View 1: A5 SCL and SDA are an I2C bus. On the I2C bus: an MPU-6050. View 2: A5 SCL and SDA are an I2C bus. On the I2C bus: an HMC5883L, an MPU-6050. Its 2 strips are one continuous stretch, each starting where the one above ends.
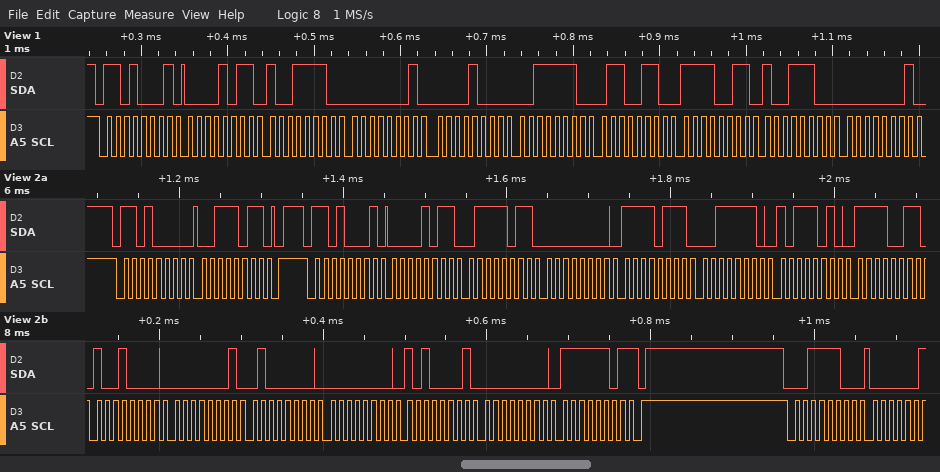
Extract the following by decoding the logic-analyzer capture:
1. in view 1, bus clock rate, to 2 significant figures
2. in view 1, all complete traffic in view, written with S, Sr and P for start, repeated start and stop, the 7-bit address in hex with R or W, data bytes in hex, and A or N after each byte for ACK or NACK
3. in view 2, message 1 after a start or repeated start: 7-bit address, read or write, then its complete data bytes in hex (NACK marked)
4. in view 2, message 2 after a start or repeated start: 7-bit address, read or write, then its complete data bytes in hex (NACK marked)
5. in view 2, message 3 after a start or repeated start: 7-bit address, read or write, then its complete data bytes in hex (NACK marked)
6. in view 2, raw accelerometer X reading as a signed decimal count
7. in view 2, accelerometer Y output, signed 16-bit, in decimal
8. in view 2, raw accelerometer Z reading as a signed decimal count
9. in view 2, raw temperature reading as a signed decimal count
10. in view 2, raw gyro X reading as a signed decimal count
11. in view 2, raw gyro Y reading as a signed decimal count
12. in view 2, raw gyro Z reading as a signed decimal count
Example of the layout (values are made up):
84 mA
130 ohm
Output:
100 kHz
S 68R A 0B A 9E A 01 A 08 A 3E A 66 A F3 A 9C A 01 A
0x68 write: 3B
0x68 read: 0B 7B 00 F7 3E BA F3 90 01 40 00 A1 00 FD NACK
0x1E write
2939
247
16058
-3184
320
161
253
